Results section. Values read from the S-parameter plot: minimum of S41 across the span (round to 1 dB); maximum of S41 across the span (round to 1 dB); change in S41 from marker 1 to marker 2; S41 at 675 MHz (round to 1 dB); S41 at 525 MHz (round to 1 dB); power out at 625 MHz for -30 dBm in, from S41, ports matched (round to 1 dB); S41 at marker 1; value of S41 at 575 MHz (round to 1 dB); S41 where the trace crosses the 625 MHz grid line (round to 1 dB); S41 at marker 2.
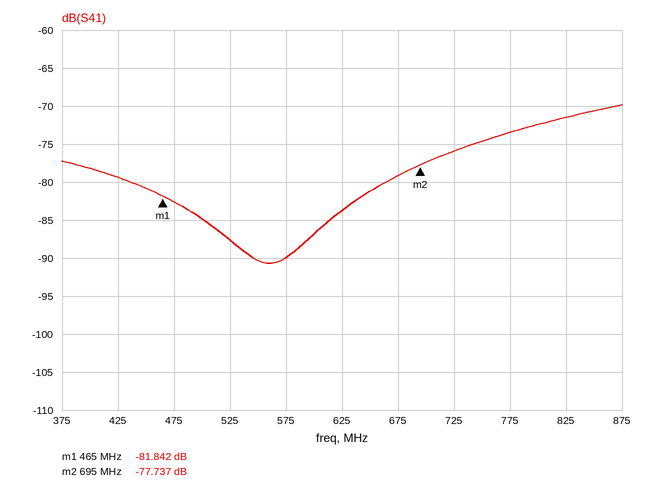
-91 dB
-70 dB
4.105 dB
-79 dB
-88 dB
-114 dBm
-81.842 dB
-90 dB
-84 dB
-77.737 dB
